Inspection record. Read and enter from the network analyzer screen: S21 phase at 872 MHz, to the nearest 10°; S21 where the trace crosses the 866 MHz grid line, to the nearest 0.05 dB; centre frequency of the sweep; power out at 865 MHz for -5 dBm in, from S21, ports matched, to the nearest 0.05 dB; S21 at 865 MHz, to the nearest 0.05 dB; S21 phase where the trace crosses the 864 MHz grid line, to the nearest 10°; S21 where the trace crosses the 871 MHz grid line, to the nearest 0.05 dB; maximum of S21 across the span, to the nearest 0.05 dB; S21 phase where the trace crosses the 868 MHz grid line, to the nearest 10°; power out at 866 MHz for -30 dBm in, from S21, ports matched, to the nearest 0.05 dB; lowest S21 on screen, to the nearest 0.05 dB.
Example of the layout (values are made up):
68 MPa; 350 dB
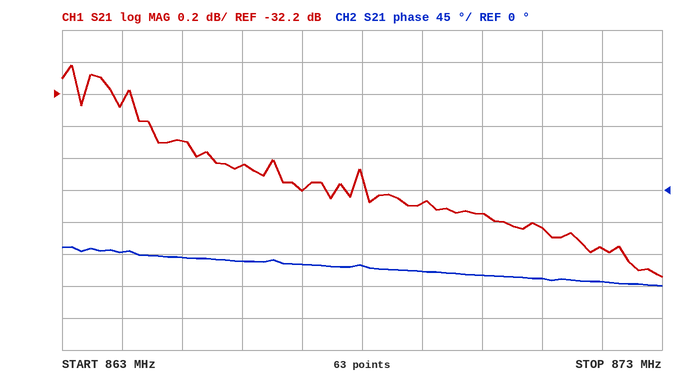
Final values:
-130°; -32.65 dB; 868 MHz; -37.50 dBm; -32.50 dB; -90°; -33.05 dB; -32.00 dB; -110°; -62.65 dBm; -33.35 dB
